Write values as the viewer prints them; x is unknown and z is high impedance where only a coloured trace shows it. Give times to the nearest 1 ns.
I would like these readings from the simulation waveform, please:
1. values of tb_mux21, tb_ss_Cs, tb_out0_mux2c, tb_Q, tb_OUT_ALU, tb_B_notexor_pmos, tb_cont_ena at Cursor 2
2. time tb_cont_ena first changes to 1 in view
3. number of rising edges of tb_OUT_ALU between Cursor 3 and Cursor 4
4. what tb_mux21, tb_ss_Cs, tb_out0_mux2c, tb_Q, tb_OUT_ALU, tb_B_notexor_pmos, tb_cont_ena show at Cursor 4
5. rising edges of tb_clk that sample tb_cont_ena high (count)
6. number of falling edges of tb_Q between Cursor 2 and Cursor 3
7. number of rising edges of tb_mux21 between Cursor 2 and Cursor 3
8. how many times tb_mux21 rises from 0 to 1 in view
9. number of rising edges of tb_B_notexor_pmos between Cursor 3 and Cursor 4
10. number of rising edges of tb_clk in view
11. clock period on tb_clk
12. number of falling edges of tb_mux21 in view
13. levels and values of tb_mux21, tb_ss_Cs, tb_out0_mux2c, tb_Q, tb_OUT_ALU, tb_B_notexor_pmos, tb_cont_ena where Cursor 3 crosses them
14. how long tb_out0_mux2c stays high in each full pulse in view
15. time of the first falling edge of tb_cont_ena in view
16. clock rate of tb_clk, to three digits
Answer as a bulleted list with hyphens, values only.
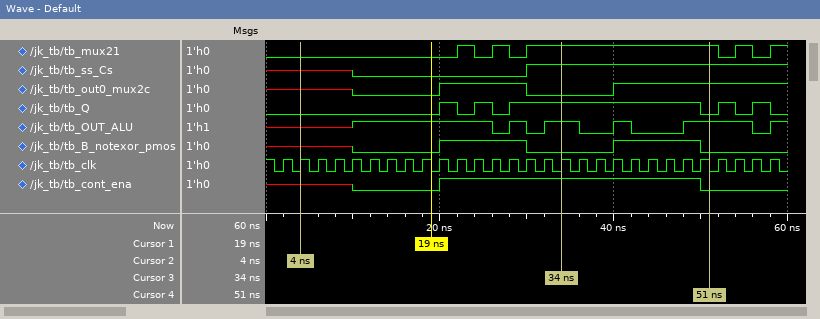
- tb_mux21=0, tb_ss_Cs=x, tb_out0_mux2c=x, tb_Q=0, tb_OUT_ALU=x, tb_B_notexor_pmos=x, tb_cont_ena=x
- 20 ns
- 2
- tb_mux21=1, tb_ss_Cs=1, tb_out0_mux2c=1, tb_Q=0, tb_OUT_ALU=1, tb_B_notexor_pmos=0, tb_cont_ena=0
- 15
- 2
- 3
- 5
- 1
- 29
- 2 ns
- 4
- tb_mux21=1, tb_ss_Cs=1, tb_out0_mux2c=0, tb_Q=1, tb_OUT_ALU=1, tb_B_notexor_pmos=0, tb_cont_ena=1
- 10 ns
- 50 ns
- 500 MHz
